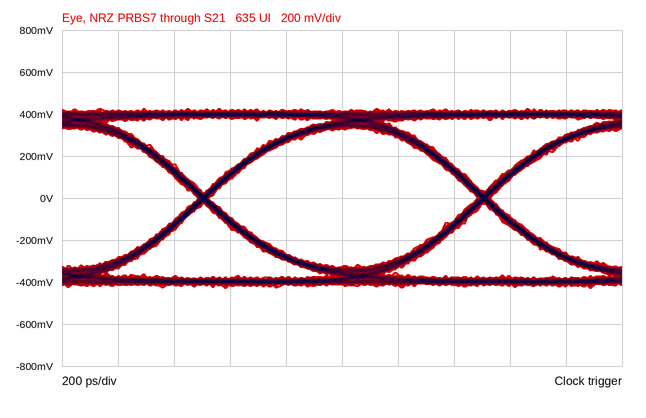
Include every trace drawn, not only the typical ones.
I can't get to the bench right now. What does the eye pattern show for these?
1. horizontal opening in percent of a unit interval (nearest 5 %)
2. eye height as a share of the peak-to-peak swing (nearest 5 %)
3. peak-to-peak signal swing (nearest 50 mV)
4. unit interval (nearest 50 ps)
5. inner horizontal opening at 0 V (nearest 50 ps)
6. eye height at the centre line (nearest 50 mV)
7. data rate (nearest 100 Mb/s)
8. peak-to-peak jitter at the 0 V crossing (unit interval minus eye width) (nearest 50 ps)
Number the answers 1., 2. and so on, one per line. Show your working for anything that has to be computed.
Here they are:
1. 950 ps / 1.00 ns ≈ 95 %
2. 650 mV / 850 mV ≈ 76.5 %, so 75 % to the nearest 5 %
3. 850 mV
4. 1.00 ns
5. 950 ps
6. 650 mV
7. 1.0 Gb/s
8. 50 ps
